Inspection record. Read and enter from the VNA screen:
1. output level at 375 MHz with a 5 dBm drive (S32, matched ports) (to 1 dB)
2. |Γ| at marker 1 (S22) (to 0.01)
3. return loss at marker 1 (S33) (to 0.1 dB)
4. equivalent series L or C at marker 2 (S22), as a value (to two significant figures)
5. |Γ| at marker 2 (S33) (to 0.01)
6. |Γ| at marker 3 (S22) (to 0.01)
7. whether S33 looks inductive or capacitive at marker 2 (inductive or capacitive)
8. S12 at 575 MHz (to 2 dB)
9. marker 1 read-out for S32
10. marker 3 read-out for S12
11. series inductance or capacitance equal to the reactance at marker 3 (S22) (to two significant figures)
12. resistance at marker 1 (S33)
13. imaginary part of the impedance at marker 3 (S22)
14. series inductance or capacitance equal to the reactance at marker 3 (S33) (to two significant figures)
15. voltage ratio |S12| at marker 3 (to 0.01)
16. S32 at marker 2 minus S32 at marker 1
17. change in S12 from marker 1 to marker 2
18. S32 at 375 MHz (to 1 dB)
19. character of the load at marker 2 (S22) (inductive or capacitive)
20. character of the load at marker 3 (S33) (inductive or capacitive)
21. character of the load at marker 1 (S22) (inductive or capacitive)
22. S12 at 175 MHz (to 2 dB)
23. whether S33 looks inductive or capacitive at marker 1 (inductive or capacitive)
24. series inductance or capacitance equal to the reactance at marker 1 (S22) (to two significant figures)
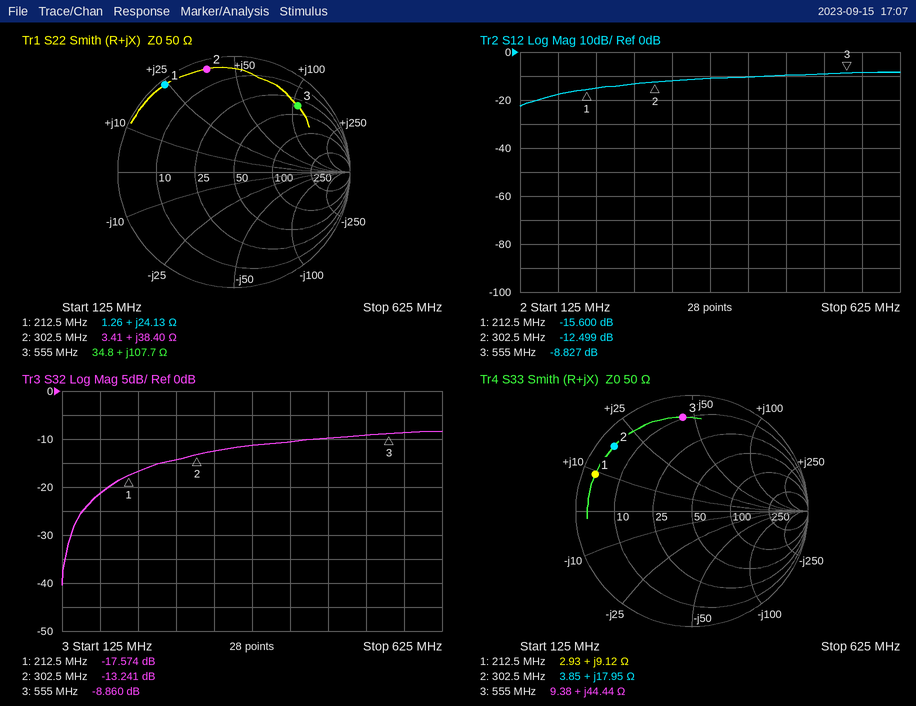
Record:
-6 dBm
0.96
1.0 dB
20 nH
0.87
0.79
inductive
-8 dB
-17.574 dB
-8.827 dB
31 nH
2.93 Ω
+107.7 Ω
13 nH
0.36
4.333 dB
3.101 dB
-11 dB
inductive
inductive
inductive
-18 dB
inductive
18 nH
